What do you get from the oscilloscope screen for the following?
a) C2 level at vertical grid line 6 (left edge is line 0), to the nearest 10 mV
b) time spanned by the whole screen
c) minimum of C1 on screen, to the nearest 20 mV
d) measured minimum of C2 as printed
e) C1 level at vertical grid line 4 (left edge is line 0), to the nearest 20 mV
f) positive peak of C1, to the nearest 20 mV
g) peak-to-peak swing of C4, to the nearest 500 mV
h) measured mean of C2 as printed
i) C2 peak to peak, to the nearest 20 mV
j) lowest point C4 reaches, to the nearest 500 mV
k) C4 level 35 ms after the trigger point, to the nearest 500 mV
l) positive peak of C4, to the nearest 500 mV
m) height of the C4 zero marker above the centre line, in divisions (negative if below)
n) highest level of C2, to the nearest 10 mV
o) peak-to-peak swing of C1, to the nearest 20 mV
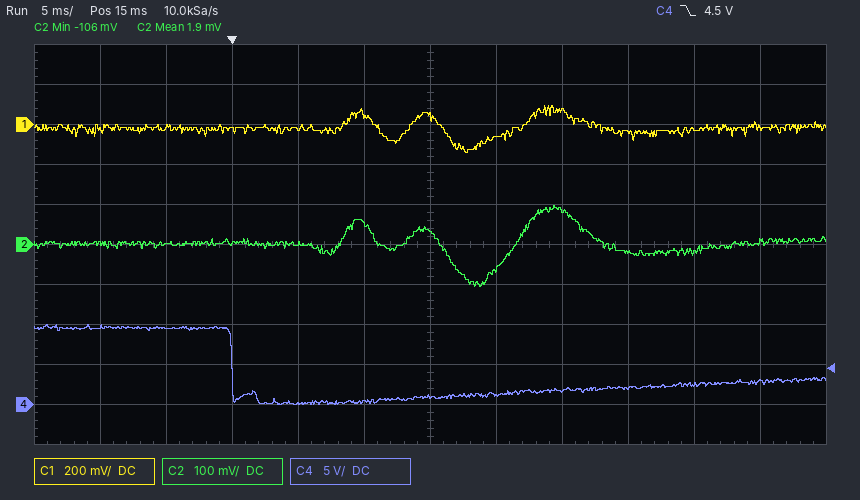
30 mV
60 ms
-140 mV
-106 mV
-20 mV
100 mV
10.0 V
1.9 mV
200 mV
0.0 V
2.5 V
10.0 V
-4.0 div
100 mV
240 mV
